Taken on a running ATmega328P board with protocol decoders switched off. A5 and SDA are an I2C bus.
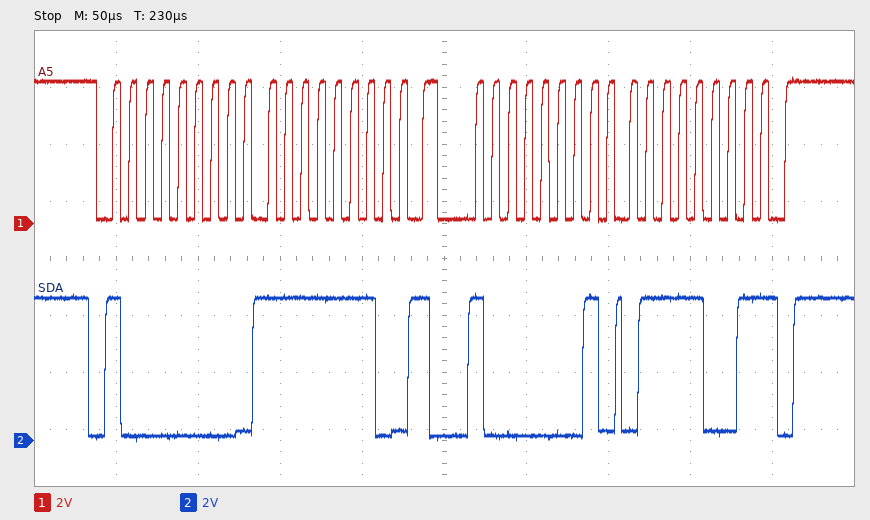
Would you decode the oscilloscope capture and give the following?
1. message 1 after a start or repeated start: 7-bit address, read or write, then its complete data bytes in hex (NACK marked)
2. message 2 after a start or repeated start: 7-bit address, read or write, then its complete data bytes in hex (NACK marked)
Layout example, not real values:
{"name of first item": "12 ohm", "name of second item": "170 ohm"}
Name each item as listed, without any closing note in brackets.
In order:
{"message 1 after a start or repeated start: 7-bit address, read or write, then its complete data bytes in hex": "0x40 write: FE", "message 2 after a start or repeated start: 7-bit address, read or write, then its complete data bytes in hex": "0x40 read: 79 NACK"}
